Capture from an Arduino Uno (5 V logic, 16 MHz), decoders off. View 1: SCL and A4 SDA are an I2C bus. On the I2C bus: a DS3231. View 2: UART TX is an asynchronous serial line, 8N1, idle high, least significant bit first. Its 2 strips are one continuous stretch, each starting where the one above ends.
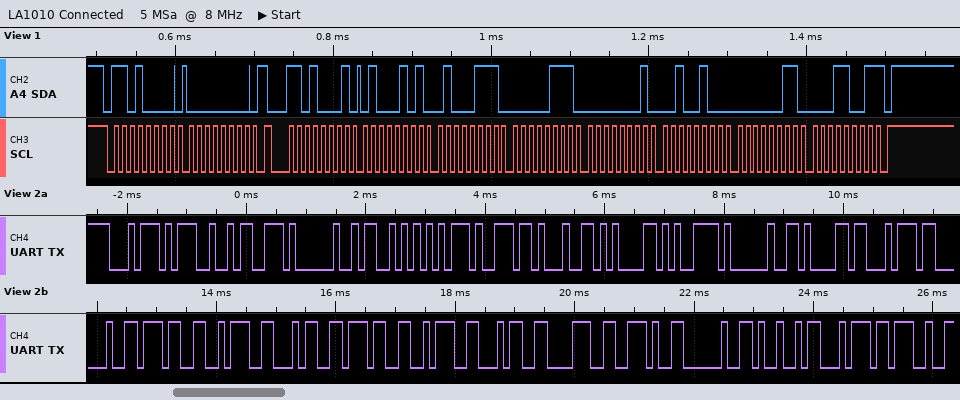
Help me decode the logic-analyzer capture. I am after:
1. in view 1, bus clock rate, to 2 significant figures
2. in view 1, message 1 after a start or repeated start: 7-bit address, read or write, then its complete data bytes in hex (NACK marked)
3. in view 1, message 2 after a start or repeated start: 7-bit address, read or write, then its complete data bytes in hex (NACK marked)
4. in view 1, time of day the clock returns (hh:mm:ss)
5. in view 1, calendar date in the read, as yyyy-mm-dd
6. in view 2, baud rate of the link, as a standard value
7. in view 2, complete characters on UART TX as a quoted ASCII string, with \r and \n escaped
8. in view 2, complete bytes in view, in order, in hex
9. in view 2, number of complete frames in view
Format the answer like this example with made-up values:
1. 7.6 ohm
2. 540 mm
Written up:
1. 100 kHz
2. 0x68 write: 00
3. 0x68 read: 45 47 07 01 24 03 19 NACK
4. 07:47:45
5. 2019-03-24
6. 9600 baud
7. "t's Sunday at 7:47:48. It'"
8. 0x74 0x27 0x73 0x20 0x53 0x75 0x6E 0x64 0x61 0x79 0x20 0x61 0x74 0x20 0x37 0x3A 0x34 0x37 0x3A 0x34 0x38 0x2E 0x20 0x49 0x74 0x27
9. 26
